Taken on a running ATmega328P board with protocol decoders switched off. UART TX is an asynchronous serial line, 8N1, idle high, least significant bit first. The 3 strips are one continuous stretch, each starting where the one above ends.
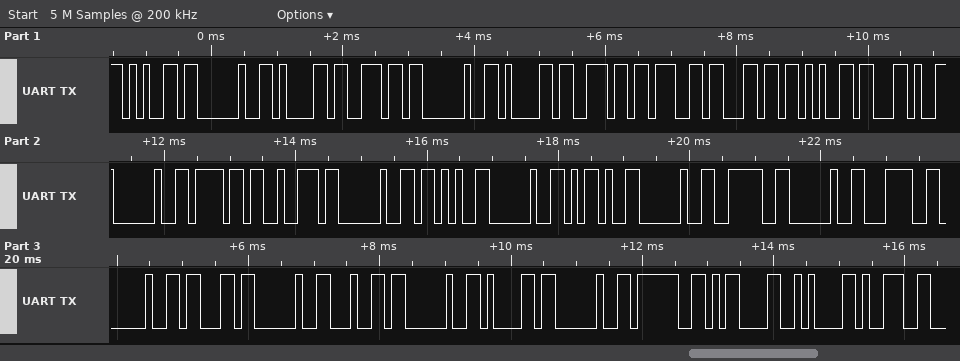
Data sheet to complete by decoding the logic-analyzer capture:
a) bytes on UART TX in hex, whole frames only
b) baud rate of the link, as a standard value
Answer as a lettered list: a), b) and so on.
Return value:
a) 65 20 61 6E 20 61 6E 67 6C 65 2C 20 6F 72 20 2B 20 2D 20 3E 20 3C 20 63 20 64 20 61 20 3F 0D 0A 39
b) 9600 baud
